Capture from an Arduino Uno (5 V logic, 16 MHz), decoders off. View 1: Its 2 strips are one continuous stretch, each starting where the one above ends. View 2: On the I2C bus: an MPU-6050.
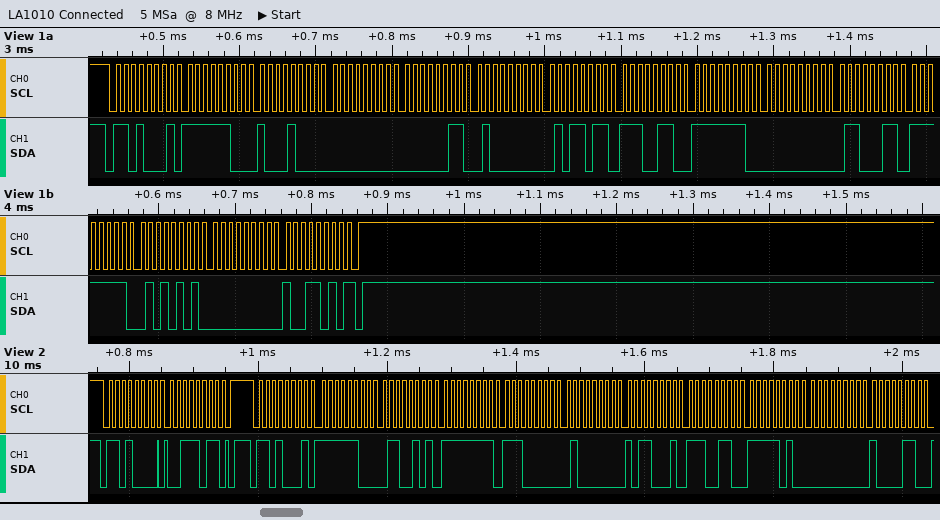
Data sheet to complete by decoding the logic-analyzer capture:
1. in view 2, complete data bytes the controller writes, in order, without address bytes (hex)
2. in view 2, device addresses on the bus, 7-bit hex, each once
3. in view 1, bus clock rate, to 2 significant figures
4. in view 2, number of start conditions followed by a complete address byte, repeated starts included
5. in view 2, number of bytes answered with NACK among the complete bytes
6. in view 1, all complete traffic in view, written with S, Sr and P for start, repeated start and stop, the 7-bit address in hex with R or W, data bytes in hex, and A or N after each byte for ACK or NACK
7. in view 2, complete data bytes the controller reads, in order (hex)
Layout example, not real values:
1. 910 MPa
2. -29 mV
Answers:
1. 3B
2. 0x68
3. 100 kHz
4. 2
5. 0
6. S 68R A FC A 88 A 00 A 03 A 40 A 5B A E6 A FE A 00 A 63 A FF A 55 A 00 A 9A N P
7. FC 65 FF E0 40 B1 E6 FA 00 86
